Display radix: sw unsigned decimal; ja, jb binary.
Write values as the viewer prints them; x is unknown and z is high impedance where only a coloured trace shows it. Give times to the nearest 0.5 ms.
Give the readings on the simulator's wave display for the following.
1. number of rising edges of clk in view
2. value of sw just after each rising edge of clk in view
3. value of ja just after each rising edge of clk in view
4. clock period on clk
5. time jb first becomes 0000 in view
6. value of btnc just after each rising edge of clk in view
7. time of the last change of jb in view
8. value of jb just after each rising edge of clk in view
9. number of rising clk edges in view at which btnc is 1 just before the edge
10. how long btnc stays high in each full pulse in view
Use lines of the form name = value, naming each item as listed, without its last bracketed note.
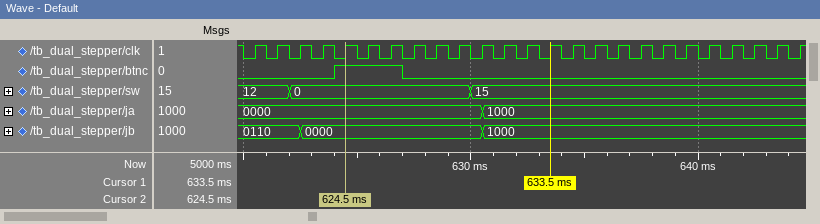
number of rising edges of clk in view = 25
value of sw just after each rising edge of clk in view = 12, 12, 0, 0, 0, 0, 0, 0, 0, 0, 15, 15, 15, 15, 15, 15, 15, 15, 15, 15, 15, 15, 15, 15, 15
value of ja just after each rising edge of clk in view = 0000, 0000, 0000, 0000, 0000, 0000, 0000, 0000, 0000, 0000, 1000, 1000, 1000, 1000, 1000, 1000, 1000, 1000, 1000, 1000, 1000, 1000, 1000, 1000, 1000
clock period on clk = 1 ms
time jb first becomes 0000 in view = 622.5 ms
value of btnc just after each rising edge of clk in view = 0 0 0 0 1 1 1 0 0 0 0 0 0 0 0 0 0 0 0 0 0 0 0 0 0
time of the last change of jb in view = 630.5 ms
value of jb just after each rising edge of clk in view = 0110, 0110, 0000, 0000, 0000, 0000, 0000, 0000, 0000, 0000, 1000, 1000, 1000, 1000, 1000, 1000, 1000, 1000, 1000, 1000, 1000, 1000, 1000, 1000, 1000
number of rising clk edges in view at which btnc is 1 just before the edge = 3
how long btnc stays high in each full pulse in view = 3 ms
